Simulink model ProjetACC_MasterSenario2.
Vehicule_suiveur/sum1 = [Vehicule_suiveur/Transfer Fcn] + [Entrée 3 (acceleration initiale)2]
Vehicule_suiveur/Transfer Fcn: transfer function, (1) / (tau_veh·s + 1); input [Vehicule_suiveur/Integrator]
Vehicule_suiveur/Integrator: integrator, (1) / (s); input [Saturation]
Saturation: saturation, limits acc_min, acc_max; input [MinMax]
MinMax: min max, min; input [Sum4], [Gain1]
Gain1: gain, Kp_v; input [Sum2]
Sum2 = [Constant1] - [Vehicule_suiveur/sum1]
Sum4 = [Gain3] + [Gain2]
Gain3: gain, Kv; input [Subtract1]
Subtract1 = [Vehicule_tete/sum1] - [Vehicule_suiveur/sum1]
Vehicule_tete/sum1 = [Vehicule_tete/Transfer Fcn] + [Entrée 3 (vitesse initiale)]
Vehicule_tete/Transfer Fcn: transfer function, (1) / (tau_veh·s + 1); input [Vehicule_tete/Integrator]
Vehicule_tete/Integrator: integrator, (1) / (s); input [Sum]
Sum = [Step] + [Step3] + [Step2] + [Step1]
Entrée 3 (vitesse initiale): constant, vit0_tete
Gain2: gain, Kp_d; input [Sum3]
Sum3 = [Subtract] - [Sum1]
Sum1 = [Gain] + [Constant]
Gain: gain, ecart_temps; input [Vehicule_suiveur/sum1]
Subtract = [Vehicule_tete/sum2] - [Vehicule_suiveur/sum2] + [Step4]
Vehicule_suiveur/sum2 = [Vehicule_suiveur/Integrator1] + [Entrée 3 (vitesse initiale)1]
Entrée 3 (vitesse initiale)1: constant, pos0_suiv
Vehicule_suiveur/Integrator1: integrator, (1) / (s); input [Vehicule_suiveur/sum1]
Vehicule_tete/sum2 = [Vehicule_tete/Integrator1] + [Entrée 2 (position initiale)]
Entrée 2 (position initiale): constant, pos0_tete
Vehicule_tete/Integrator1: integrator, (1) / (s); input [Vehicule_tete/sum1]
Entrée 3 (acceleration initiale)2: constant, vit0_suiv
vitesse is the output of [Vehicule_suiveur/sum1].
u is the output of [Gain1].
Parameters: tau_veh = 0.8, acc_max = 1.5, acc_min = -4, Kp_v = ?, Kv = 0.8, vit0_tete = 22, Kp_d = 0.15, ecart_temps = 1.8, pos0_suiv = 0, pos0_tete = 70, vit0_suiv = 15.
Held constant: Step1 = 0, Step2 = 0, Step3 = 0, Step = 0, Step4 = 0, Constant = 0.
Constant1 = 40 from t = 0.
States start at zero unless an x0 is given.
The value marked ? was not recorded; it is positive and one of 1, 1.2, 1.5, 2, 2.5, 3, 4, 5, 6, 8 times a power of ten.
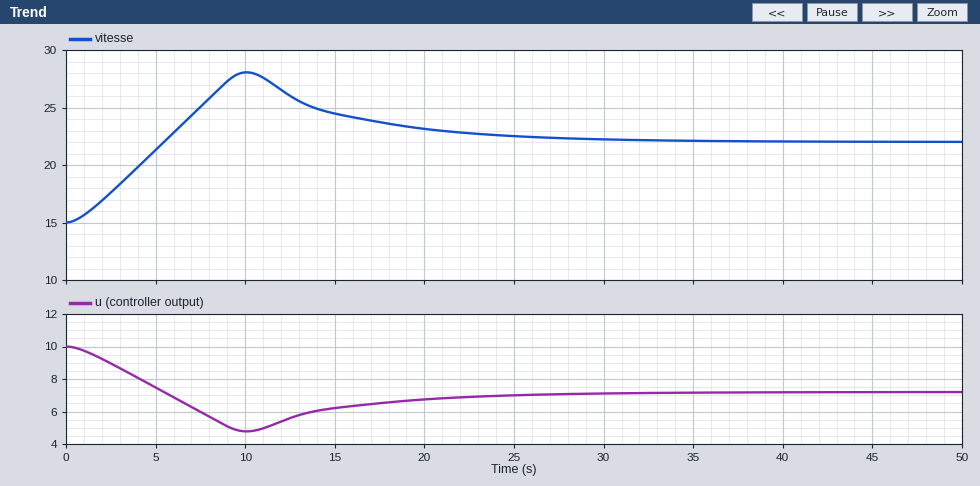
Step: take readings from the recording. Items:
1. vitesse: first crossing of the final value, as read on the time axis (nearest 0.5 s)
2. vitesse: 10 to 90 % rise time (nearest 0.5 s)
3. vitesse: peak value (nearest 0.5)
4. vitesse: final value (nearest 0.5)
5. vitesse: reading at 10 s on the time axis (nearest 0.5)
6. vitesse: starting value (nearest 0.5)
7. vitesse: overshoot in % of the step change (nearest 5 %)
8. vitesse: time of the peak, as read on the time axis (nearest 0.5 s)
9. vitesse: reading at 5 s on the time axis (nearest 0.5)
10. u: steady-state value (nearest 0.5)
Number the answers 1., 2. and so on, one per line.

1. 5.5 s
2. 4.0 s
3. 28.0
4. 22.0
5. 28.0
6. 15.0
7. 85 %
8. 10.0 s
9. 21.5
10. 7.0
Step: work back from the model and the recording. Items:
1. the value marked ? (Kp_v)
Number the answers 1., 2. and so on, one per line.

1. 0.4
